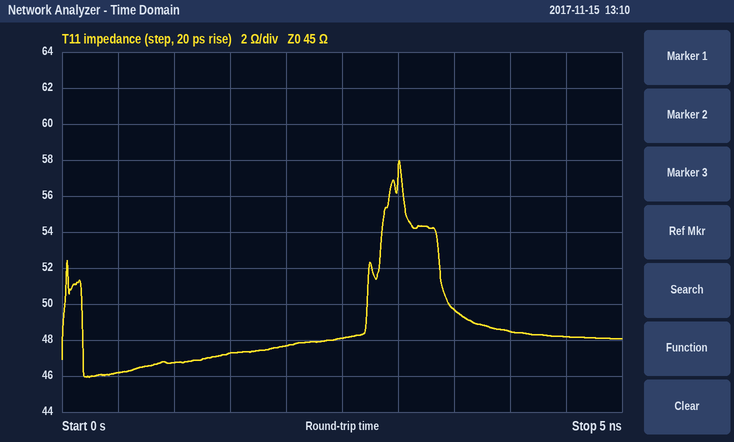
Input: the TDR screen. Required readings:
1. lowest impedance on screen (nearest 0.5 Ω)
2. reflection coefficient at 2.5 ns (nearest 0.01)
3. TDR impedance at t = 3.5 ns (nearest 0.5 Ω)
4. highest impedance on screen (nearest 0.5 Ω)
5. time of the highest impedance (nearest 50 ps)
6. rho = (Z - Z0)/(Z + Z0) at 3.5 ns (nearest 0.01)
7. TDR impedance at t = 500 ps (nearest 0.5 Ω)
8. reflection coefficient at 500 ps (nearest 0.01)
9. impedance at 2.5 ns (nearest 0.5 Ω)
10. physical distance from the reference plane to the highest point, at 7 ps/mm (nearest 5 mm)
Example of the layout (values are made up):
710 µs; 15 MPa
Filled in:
46.0 Ω; +0.03; 49.5 Ω; 58.0 Ω; 3.00 ns; +0.05; 46.0 Ω; +0.01; 48.0 Ω; 215 mm
